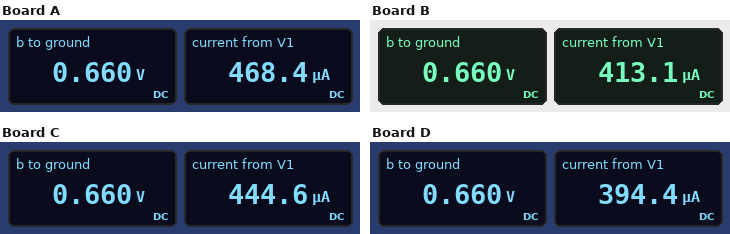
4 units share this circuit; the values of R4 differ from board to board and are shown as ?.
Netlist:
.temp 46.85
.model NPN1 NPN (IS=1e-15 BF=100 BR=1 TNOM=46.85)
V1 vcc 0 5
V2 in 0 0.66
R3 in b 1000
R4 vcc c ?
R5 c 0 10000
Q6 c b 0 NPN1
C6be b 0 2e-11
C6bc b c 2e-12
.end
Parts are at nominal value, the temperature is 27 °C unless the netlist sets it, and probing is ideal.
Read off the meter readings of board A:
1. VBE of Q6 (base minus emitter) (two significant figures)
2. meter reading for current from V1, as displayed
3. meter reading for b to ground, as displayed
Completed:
660 mV
468.4 µA
0.660 V
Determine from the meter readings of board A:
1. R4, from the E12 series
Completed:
1.2 kΩ
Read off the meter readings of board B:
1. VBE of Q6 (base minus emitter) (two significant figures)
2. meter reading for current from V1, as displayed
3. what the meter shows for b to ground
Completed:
660 mV
413.1 µA
0.660 V
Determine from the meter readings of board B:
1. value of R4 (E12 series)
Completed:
2.7 kΩ
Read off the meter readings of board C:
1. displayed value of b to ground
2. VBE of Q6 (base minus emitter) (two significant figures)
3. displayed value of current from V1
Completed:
0.660 V
660 mV
444.6 µA
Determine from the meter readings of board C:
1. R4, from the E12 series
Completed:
1.8 kΩ
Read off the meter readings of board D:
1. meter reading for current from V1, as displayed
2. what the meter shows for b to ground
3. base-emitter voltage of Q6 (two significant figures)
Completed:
394.4 µA
0.660 V
660 mV
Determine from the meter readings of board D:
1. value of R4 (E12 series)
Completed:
3.3 kΩ
